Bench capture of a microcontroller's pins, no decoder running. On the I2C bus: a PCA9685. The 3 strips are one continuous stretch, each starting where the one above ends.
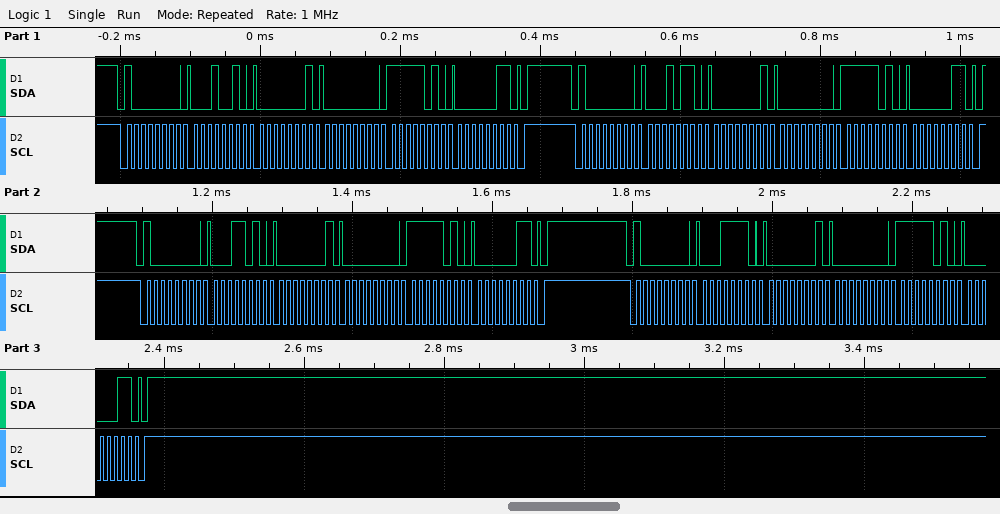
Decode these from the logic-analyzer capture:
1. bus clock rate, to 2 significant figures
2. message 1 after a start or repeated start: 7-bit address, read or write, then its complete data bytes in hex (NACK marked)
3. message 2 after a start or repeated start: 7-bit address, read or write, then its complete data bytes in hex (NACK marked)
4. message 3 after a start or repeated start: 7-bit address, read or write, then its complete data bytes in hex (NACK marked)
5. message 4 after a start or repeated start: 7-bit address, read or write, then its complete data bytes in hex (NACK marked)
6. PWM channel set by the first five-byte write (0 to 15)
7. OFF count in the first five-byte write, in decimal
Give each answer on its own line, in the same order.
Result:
100 kHz
0x40 write: 12 01 00 FA 03
0x40 write: 16 01 00 FA 03
0x40 write: 1A 01 00 FA 03
0x40 write: 1E 01 00 FA 03
3
1018
